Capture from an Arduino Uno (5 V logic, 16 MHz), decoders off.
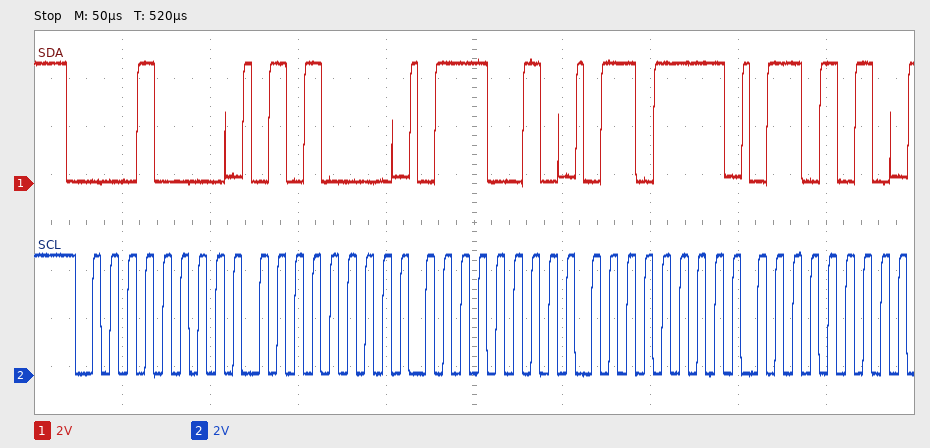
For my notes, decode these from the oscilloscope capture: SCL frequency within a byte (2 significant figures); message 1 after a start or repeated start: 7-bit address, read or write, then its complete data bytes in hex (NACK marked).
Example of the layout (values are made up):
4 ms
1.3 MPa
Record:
100 kHz
0x08 write: 50 72 6F 6A
